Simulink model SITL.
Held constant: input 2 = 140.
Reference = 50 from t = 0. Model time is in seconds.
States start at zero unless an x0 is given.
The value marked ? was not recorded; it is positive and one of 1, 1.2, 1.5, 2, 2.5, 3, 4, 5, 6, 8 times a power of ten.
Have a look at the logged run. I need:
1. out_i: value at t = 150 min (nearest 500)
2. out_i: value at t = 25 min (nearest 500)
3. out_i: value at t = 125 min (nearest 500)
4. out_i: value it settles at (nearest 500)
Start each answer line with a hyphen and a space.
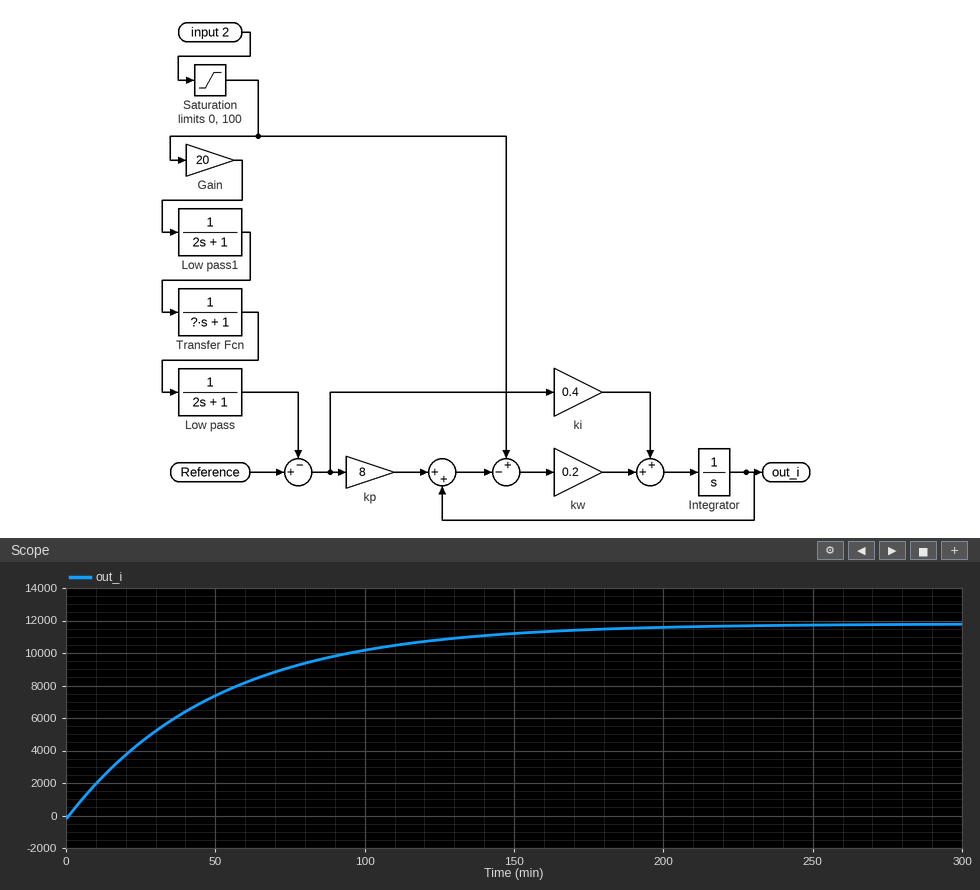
- 11000
- 4500
- 11000
- 12000
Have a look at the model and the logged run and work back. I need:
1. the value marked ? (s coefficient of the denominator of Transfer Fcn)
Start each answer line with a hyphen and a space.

- 3000
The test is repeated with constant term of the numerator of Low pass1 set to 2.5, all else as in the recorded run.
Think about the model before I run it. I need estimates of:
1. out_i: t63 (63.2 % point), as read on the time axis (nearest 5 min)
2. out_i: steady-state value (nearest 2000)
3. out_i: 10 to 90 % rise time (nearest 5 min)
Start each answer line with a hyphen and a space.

- 50 min
- 30000
- 110 min
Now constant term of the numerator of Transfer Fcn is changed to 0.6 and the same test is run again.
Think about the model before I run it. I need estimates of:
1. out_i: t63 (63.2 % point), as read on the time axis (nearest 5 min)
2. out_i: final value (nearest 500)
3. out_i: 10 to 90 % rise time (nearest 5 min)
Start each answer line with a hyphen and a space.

- 50 min
- 7000
- 110 min
